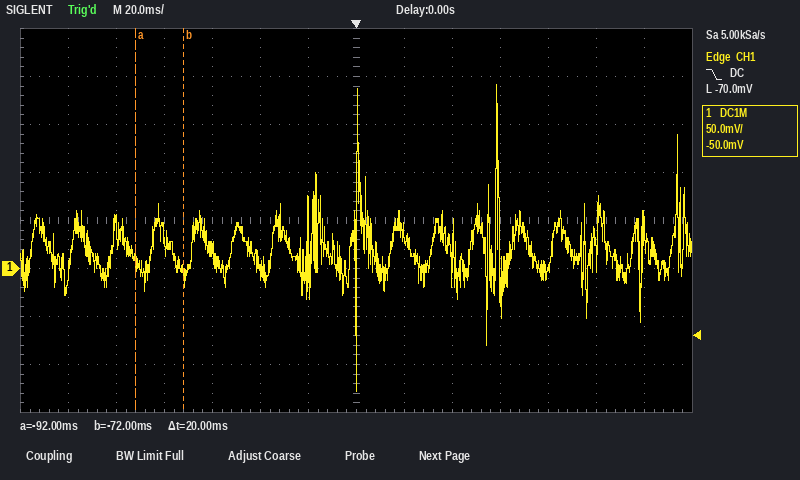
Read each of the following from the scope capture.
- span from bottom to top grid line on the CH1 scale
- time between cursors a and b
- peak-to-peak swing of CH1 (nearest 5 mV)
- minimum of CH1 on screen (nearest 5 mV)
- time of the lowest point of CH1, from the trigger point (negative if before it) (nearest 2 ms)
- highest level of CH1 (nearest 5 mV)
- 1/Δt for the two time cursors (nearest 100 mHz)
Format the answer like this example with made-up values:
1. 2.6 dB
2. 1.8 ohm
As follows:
1. 400 mV
2. 20 ms
3. 320 mV
4. -130 mV
5. 0 ms
6. 190 mV
7. 50.0 Hz
